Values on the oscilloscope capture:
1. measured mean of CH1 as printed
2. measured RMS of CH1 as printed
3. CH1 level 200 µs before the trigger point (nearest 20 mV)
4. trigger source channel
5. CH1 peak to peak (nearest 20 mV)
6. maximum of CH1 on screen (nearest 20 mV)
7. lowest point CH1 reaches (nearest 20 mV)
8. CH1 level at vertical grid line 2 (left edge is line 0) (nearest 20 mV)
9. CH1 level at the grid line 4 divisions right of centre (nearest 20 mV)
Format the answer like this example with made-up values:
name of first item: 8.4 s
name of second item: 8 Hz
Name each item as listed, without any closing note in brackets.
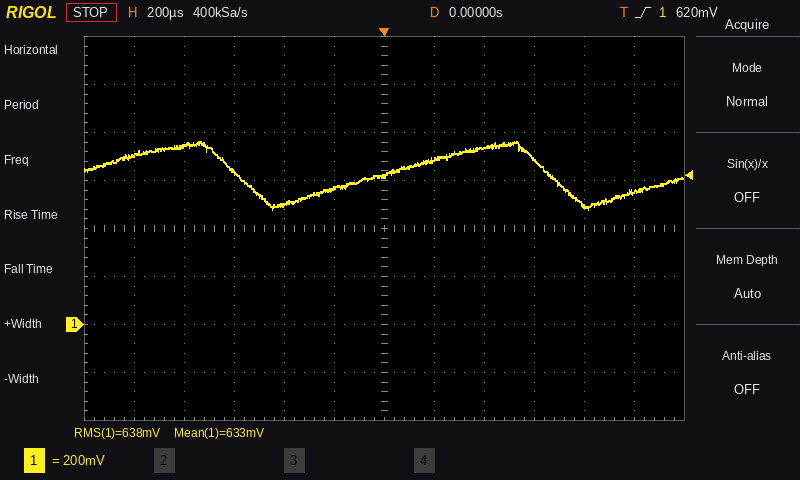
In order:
measured mean of CH1 as printed: 633 mV
measured RMS of CH1 as printed: 638 mV
CH1 level 200 µs before the trigger point: 560 mV
trigger source channel: CH1
CH1 peak to peak: 280 mV
maximum of CH1 on screen: 760 mV
lowest point CH1 reaches: 480 mV
CH1 level at vertical grid line 2 (left edge is line 0): 740 mV
CH1 level at the grid line 4 divisions right of centre: 500 mV
